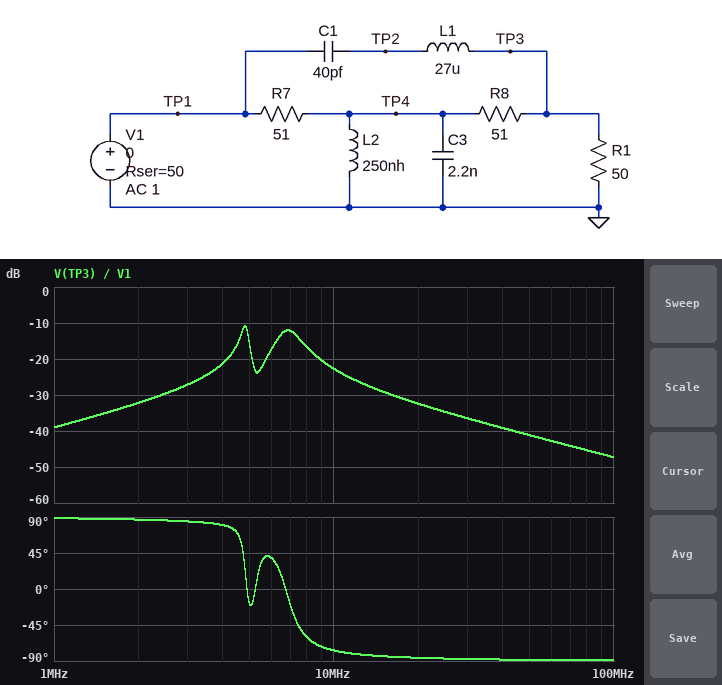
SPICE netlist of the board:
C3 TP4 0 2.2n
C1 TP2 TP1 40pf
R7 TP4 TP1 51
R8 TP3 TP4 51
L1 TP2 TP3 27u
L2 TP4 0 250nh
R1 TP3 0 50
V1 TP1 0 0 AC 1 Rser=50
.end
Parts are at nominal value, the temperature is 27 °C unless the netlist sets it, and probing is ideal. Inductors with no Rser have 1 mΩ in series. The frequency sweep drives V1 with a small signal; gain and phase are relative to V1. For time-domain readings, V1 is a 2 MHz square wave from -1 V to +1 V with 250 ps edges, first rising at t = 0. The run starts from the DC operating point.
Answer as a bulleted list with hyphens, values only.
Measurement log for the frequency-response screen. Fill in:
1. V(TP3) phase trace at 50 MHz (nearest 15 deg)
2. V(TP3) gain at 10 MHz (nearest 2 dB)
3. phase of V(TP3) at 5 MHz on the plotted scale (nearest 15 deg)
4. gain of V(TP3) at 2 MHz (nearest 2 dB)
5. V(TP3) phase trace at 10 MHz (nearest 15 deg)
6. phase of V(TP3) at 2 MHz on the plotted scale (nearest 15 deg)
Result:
- -90 deg
- -22 dB
- -15 deg
- -32 dB
- -75 deg
- 90 deg
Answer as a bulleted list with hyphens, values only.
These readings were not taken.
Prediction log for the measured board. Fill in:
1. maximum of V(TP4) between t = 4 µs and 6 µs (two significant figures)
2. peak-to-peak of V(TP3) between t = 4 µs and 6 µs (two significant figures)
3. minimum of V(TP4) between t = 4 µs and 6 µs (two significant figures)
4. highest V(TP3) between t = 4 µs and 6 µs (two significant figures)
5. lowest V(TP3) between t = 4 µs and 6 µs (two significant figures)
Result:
- 200 mV
- 210 mV
- -200 mV
- 110 mV
- -110 mV
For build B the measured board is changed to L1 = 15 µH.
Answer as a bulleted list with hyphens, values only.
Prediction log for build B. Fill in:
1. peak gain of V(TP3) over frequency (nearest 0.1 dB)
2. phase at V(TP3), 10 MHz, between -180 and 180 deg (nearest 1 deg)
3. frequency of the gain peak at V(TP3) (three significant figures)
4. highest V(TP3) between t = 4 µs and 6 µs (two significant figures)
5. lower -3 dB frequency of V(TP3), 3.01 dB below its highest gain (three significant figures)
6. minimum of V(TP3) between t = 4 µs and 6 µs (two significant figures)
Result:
- -6.5 dB
- -78 deg
- 6.50 MHz
- 160 mV
- 6.16 MHz
- -160 mV
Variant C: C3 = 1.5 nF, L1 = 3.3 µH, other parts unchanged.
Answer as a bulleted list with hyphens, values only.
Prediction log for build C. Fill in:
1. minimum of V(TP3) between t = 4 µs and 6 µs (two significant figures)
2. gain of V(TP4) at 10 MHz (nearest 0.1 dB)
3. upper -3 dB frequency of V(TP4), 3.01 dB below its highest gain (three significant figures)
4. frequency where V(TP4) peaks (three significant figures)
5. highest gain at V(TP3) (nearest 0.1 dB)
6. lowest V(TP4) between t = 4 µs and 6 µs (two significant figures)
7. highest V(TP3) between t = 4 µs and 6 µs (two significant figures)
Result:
- -170 mV
- -11.3 dB
- 9.34 MHz
- 8.22 MHz
- -11.2 dB
- -180 mV
- 170 mV
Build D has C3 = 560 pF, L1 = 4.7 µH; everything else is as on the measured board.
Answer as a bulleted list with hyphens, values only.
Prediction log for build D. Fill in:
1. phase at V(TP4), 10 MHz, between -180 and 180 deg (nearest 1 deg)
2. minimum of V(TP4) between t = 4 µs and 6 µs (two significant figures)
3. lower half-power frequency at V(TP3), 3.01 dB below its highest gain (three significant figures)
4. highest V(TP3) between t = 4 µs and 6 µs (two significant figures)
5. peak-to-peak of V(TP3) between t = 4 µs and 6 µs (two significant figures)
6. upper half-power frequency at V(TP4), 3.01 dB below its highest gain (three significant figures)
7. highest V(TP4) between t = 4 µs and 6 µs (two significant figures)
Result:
- 55 deg
- -310 mV
- 10.5 MHz
- 210 mV
- 420 mV
- 16.6 MHz
- 310 mV
